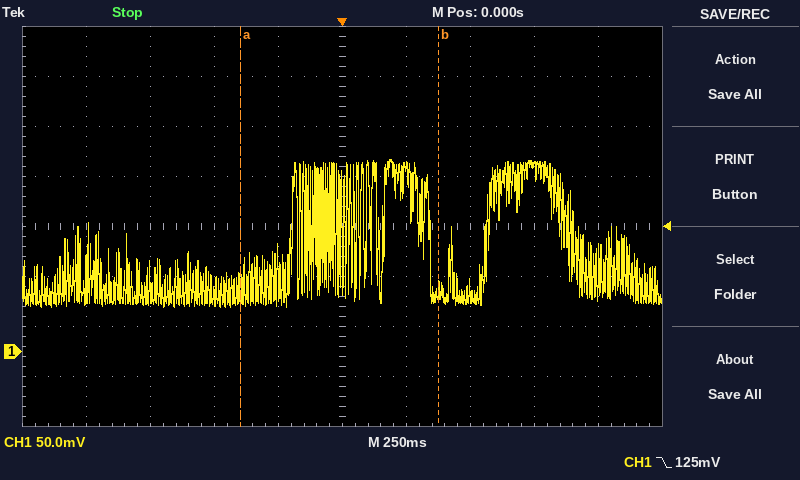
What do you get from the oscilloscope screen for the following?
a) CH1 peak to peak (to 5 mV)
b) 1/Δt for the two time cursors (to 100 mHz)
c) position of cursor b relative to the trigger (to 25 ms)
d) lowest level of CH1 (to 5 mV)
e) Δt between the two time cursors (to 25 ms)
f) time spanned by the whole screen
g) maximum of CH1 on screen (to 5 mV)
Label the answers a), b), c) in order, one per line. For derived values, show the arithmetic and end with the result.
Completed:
a) 190 mV − (45 mV) = 145 mV
b) 1 / 775 ms ≈ 1.3 Hz
c) +375 ms
d) 45 mV
e) 775 ms
f) 2.5 s
g) 190 mV
